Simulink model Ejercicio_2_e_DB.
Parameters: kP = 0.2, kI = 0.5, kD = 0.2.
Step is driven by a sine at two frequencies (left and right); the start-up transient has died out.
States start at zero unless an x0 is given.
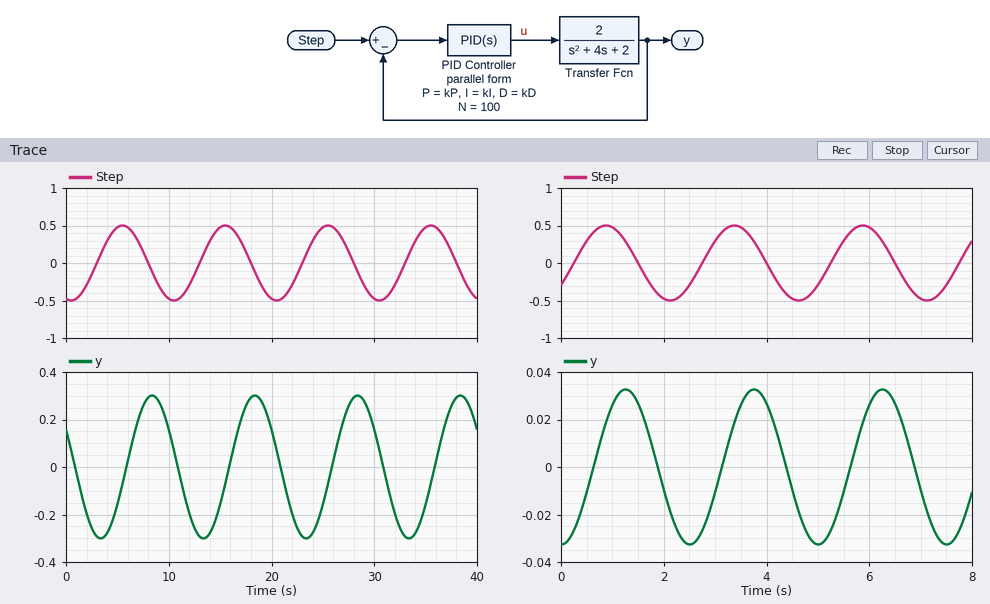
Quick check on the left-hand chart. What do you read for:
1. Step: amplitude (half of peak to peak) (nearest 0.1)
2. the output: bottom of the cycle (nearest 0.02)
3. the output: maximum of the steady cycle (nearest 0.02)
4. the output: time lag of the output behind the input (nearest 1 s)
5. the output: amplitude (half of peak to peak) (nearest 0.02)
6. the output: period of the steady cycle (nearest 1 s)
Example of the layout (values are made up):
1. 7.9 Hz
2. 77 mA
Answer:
1. 0.5
2. -0.30
3. 0.30
4. 3 s
5. 0.30
6. 10 s
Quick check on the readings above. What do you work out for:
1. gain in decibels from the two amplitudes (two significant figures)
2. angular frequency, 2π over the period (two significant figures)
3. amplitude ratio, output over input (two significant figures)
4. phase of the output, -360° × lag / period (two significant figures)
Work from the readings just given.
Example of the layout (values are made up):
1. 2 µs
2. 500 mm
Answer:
1. -4.4 dB
2. 0.63 rad/s
3. 0.60
4. -110°
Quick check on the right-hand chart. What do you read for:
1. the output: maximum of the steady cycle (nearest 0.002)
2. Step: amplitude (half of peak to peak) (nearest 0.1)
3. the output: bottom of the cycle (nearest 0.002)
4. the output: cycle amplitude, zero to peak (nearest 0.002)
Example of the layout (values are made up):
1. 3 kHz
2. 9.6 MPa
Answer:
1. 0.032
2. 0.5
3. -0.032
4. 0.032
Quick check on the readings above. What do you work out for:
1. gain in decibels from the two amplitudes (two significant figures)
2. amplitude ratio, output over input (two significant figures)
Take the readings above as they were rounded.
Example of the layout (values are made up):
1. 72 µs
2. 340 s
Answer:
1. -24 dB
2. 0.064
